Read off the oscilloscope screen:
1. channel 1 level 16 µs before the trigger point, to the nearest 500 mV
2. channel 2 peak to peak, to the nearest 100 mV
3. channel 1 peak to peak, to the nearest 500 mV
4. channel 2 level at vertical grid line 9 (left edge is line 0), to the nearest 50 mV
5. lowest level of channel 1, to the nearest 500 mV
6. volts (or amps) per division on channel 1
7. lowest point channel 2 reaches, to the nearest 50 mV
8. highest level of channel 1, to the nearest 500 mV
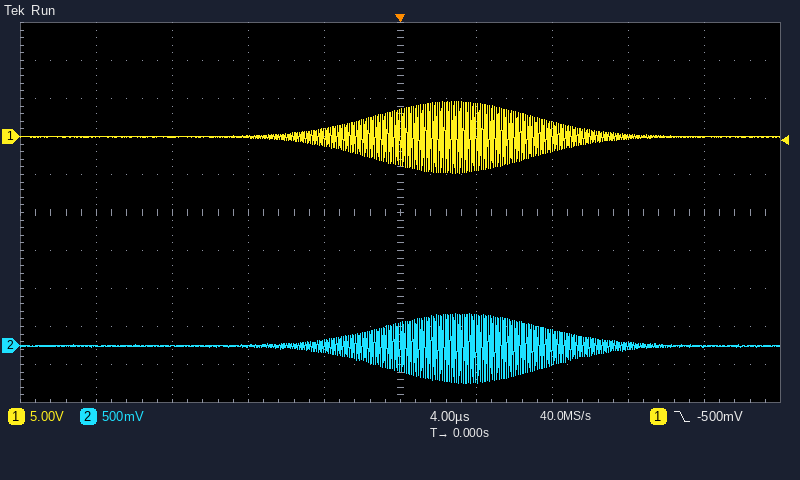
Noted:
0.0 V
900 mV
9.5 V
0 mV
-5.0 V
5 V
-500 mV
4.5 V
